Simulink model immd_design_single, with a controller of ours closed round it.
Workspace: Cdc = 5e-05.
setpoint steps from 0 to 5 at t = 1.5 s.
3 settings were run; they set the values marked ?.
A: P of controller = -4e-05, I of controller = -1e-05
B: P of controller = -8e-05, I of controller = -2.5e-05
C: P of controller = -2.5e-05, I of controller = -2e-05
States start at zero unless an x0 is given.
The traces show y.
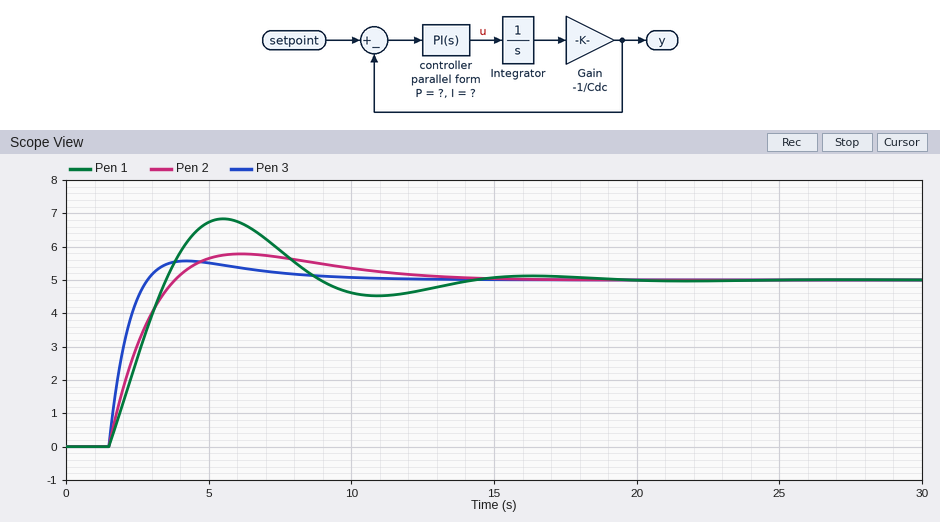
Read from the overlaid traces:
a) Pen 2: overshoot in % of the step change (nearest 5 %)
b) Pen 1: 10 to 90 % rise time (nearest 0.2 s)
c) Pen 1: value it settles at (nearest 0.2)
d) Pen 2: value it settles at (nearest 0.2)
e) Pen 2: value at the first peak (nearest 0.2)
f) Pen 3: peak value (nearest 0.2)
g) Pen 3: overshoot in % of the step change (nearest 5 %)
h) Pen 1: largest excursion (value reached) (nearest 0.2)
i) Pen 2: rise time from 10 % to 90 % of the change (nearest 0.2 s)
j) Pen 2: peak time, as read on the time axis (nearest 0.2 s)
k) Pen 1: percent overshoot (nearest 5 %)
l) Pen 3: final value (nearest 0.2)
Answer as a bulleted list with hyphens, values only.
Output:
- 15 %
- 1.6 s
- 5.0
- 5.0
- 5.8
- 5.6
- 10 %
- 6.8
- 1.8 s
- 6.2 s
- 35 %
- 5.0
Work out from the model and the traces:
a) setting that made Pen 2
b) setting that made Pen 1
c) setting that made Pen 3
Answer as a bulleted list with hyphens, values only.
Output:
- A
- C
- B
